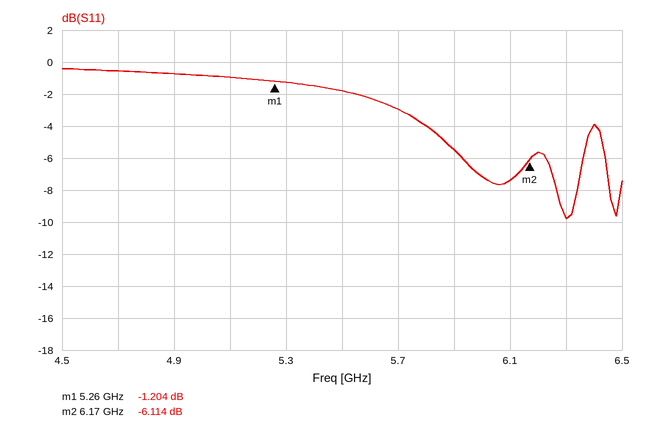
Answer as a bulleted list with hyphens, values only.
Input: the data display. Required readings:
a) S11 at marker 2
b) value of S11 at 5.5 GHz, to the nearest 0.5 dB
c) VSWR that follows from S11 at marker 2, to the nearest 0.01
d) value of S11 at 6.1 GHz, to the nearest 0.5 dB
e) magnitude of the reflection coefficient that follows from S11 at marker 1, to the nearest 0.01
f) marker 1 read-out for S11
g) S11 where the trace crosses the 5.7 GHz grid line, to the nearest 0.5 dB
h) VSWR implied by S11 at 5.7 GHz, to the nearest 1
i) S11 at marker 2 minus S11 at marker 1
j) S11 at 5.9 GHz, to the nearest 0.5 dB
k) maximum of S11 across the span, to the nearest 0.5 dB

- -6.114 dB
- -2.0 dB
- 2.96
- -7.5 dB
- 0.87
- -1.204 dB
- -3.0 dB
- 6
- -4.910 dB
- -5.5 dB
- -0.5 dB
